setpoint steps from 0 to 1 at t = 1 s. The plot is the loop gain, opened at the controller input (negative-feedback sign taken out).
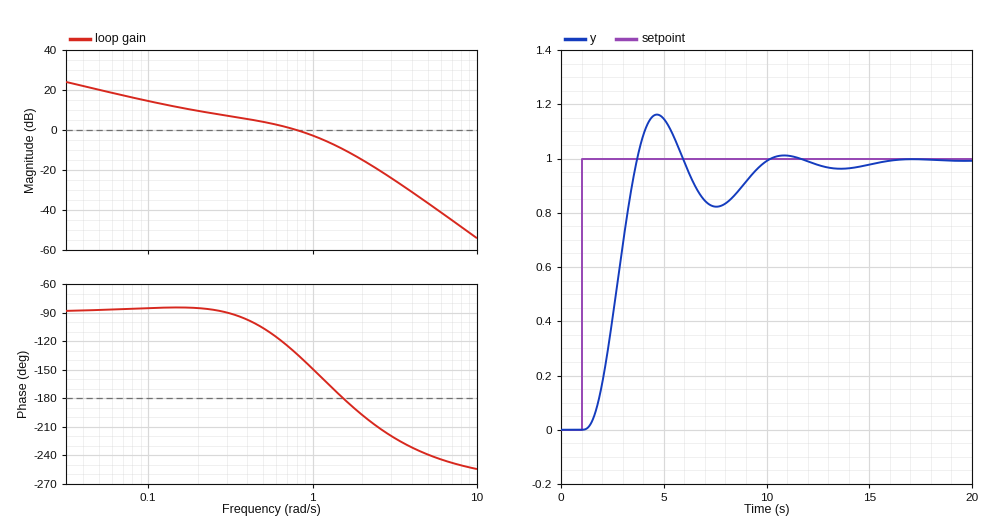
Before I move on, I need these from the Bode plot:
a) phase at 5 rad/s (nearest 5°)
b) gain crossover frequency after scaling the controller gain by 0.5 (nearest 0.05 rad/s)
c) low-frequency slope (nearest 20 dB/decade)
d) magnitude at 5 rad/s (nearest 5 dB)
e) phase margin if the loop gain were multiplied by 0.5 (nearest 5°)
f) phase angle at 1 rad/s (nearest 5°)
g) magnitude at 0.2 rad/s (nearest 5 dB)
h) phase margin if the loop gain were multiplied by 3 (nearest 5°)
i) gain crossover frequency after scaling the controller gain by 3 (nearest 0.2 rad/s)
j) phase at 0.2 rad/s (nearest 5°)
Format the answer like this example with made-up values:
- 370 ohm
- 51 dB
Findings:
- -240°
- 0.35 rad/s
- -20 dB/decade
- -35 dB
- 85°
- -150°
- 10 dB
- 0°
- 1.6 rad/s
- -85°
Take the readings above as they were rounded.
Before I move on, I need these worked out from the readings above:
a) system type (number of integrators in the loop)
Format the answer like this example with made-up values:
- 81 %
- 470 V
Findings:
- 1
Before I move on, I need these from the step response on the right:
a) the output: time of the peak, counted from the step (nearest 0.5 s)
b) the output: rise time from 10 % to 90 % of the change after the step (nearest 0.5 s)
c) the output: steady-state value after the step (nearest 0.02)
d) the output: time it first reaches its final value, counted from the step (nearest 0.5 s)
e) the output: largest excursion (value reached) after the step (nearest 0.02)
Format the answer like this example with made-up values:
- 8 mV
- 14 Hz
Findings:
- 3.5 s
- 1.5 s
- 1.00
- 2.5 s
- 1.16
